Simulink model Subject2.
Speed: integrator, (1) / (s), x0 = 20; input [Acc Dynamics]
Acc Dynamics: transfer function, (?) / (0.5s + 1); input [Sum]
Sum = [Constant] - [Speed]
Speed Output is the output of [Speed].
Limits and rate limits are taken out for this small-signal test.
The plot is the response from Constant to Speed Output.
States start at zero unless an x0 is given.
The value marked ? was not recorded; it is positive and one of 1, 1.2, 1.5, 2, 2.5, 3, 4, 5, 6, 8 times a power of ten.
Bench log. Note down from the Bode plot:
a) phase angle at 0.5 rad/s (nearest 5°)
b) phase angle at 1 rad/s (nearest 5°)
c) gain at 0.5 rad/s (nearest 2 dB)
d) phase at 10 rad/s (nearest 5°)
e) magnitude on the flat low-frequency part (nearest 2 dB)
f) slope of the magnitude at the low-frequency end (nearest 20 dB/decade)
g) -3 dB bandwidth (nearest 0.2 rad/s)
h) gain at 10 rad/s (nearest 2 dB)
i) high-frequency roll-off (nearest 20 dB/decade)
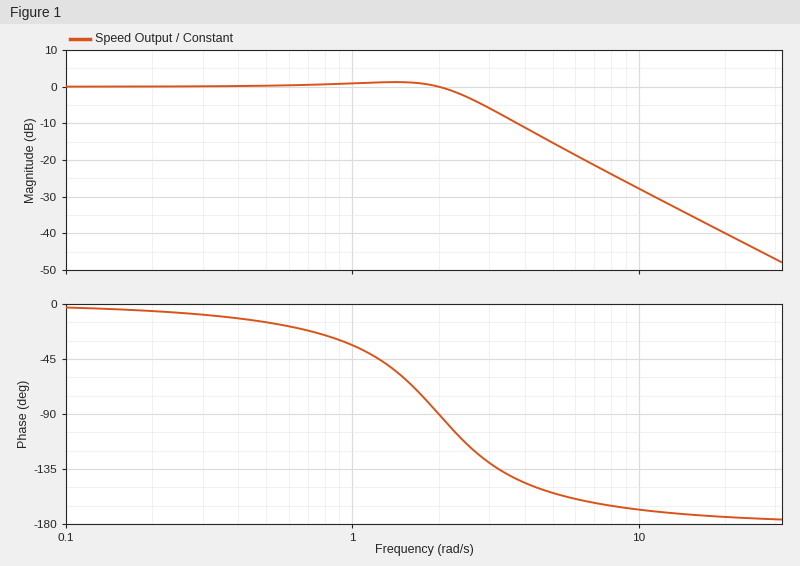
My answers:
-15°
-35°
0 dB
-170°
0 dB
0 dB/decade
2.6 rad/s
-28 dB
-40 dB/decade
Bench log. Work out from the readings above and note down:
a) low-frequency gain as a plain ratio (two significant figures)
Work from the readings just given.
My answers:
1.0
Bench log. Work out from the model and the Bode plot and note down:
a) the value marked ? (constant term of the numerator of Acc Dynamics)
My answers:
2
